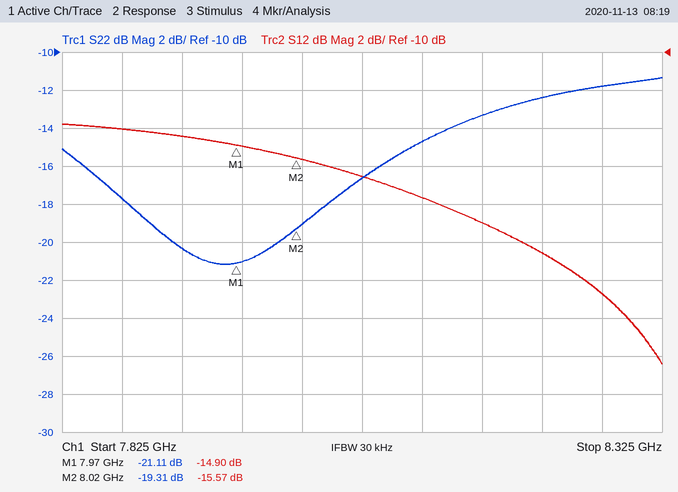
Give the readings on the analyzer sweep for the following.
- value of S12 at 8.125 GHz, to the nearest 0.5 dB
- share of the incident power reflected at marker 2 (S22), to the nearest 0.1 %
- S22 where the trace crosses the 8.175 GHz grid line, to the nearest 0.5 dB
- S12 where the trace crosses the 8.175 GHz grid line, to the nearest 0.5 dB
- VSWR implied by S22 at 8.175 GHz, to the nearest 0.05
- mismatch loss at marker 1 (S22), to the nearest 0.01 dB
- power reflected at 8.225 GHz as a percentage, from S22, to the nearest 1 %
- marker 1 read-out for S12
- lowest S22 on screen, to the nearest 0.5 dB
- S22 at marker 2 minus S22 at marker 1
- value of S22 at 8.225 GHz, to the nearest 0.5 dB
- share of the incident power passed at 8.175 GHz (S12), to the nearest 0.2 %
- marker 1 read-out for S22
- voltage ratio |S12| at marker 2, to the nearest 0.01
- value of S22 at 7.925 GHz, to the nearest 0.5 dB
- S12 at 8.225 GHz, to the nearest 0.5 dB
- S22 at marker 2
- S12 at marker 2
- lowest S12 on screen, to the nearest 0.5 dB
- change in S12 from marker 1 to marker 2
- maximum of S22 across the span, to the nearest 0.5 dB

-17.5 dB
1.2 %
-13.5 dB
-19.0 dB
1.55
0.03 dB
6 %
-14.90 dB
-21.0 dB
1.80 dB
-12.5 dB
1.2 %
-21.11 dB
0.17
-20.5 dB
-20.5 dB
-19.31 dB
-15.57 dB
-26.5 dB
-0.67 dB
-11.5 dB
